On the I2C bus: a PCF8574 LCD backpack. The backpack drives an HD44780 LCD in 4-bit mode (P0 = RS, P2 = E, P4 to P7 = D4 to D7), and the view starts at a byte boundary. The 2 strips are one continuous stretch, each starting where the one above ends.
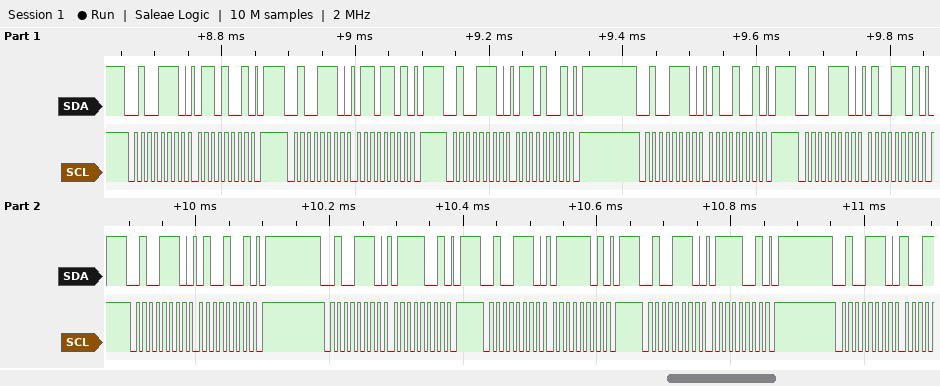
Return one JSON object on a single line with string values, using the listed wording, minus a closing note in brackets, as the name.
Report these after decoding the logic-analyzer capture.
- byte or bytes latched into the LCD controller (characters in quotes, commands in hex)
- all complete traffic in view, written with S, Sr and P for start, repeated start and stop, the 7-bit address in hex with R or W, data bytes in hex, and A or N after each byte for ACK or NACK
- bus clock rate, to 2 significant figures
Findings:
{"byte or bytes latched into the LCD controller": "'d'", "all complete traffic in view, written with S, Sr and P for start, repeated start and stop, the 7-bit address in hex with R or W, data bytes in hex, and A or N after each byte for ACK or NACK": "S 27W A 69 A P S 27W A 6D A P S 27W A 69 A P S 27W A 49 A P S 27W A 4D A P S 27W A 49 A P S 27W A 79 A P S 27W A 7D A P S 27W A 79 A P S 27W A", "bus clock rate, to 2 significant figures": "100 kHz"}
